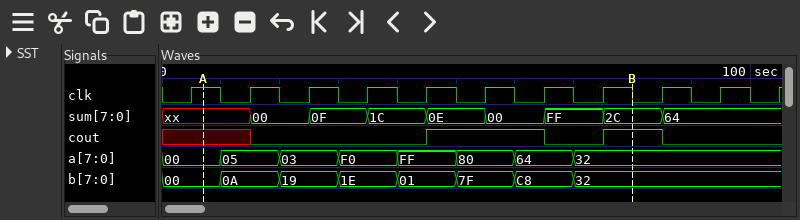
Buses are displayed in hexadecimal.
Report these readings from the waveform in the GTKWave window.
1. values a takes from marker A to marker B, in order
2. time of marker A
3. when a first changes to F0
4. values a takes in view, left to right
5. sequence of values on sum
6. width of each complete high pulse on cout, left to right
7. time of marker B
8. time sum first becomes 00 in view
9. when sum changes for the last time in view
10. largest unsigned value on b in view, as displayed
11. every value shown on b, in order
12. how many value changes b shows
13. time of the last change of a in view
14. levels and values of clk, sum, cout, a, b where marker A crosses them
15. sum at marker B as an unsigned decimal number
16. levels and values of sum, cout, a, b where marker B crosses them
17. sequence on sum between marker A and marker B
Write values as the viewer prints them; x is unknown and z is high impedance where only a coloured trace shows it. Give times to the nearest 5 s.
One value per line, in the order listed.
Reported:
00, 05, 03, F0, FF, 80, 64, 32
5 s
30 s
00, 05, 03, F0, FF, 80, 64, 32
xx, 00, 0F, 1C, 0E, 00, FF, 2C, 64
20 s, 10 s
80 s
15 s
85 s
C8
00, 0A, 19, 1E, 01, 7F, C8, 32
7
70 s
clk=1, sum=xx, cout=x, a=00, b=00
44
sum=2C, cout=1, a=32, b=32
xx, 00, 0F, 1C, 0E, 00, FF, 2C
